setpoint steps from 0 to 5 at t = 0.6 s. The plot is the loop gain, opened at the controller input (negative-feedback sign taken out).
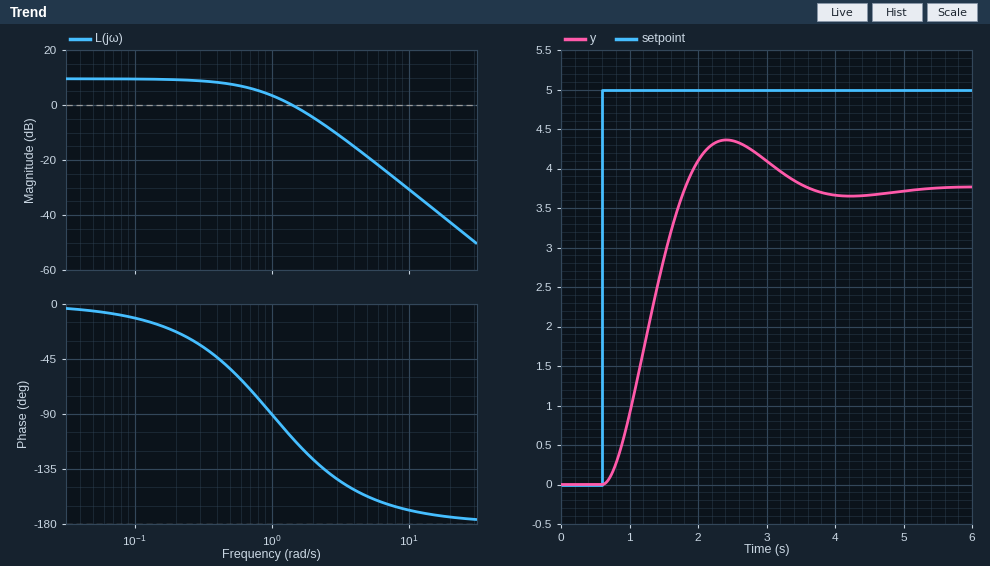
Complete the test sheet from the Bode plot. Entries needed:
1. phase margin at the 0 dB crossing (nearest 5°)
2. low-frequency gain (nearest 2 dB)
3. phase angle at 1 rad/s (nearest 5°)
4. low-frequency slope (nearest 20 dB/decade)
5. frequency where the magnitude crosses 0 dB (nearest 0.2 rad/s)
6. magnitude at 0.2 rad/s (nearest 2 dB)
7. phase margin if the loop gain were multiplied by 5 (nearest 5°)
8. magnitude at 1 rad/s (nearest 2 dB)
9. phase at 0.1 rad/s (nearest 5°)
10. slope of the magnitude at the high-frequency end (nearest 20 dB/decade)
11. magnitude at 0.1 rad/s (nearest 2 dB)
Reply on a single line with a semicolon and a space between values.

70°; 10 dB; -90°; 0 dB/decade; 1.4 rad/s; 10 dB; 30°; 4 dB; -10°; -40 dB/decade; 10 dB
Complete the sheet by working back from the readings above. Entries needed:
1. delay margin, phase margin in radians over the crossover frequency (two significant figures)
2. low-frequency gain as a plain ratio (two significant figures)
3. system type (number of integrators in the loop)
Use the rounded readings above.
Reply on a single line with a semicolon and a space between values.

0.87 s; 3.2; 0
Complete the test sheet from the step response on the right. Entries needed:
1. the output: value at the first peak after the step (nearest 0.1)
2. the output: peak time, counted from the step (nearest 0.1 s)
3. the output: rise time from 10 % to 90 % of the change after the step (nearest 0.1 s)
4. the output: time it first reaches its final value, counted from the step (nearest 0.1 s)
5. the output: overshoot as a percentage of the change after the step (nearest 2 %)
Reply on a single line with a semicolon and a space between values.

4.4; 1.8 s; 0.8 s; 1.2 s; 16 %
